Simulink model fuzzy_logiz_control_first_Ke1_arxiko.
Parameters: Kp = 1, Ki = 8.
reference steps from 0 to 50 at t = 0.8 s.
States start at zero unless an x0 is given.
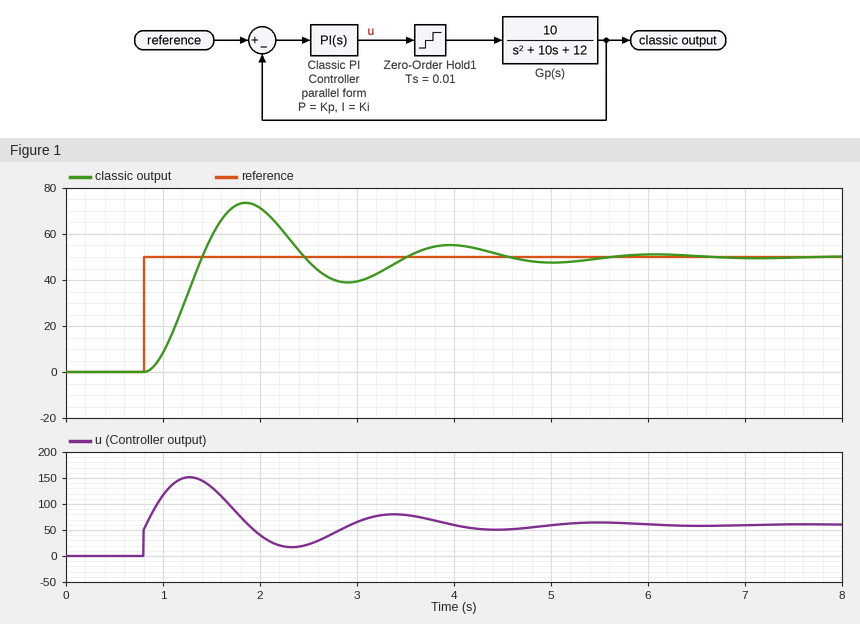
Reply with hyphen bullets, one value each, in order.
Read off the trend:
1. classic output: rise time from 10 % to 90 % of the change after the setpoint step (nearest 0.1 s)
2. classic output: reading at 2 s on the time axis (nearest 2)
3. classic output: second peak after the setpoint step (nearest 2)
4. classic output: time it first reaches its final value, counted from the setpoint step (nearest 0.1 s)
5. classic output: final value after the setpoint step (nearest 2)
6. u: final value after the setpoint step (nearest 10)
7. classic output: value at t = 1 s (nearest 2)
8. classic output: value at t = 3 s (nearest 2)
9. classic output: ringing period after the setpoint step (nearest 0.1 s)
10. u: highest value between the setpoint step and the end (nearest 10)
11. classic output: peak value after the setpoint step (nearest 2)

- 0.4 s
- 72
- 56
- 0.6 s
- 50
- 60
- 8
- 40
- 2.1 s
- 150
- 74
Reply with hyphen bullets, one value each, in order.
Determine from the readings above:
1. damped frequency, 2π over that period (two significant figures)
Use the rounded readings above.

- 3.0 rad/s
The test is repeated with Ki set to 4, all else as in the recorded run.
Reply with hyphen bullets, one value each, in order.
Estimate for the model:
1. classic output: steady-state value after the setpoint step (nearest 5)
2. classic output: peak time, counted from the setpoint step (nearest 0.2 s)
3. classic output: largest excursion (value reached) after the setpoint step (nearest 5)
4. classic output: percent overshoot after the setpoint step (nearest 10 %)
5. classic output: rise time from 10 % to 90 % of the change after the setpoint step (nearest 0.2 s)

- 50
- 1.4 s
- 60
- 20 %
- 0.6 s
